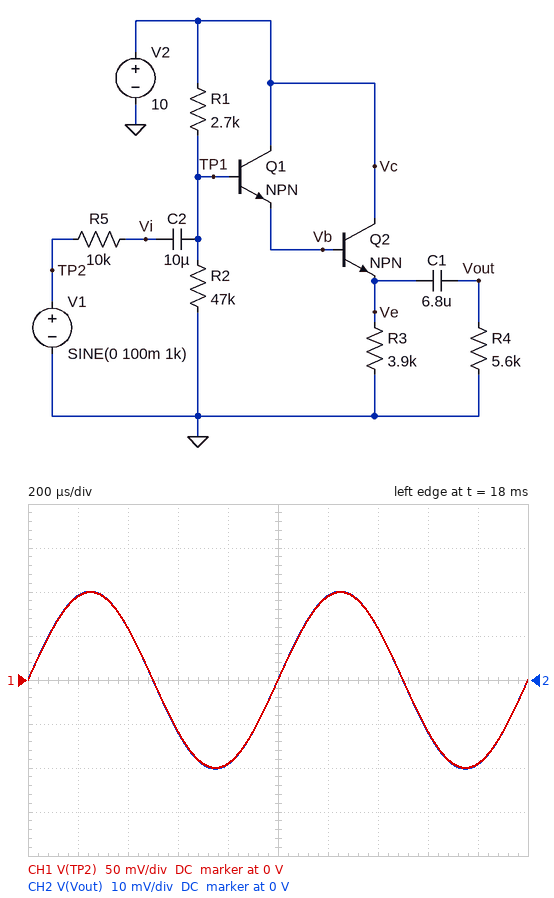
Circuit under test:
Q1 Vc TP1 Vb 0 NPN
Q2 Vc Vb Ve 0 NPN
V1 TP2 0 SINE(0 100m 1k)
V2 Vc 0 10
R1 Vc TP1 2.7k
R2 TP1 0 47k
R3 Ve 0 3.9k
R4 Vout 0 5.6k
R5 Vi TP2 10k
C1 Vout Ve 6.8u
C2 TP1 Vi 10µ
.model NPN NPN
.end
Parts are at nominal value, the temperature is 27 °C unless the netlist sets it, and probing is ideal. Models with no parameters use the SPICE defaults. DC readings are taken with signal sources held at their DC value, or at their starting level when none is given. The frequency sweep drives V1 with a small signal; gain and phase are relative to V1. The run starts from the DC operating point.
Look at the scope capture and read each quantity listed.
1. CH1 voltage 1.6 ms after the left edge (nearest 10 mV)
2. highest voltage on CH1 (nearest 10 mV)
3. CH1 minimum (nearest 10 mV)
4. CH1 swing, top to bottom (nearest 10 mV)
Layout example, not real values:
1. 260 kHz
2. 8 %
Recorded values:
1. -60 mV
2. 100 mV
3. -100 mV
4. 200 mV
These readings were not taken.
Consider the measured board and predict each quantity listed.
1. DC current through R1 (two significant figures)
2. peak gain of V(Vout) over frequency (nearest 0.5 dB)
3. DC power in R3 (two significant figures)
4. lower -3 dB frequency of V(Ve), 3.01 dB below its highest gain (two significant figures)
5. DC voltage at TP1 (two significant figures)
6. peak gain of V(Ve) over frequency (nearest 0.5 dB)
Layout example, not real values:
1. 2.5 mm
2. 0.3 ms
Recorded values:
1. 200 µA
2. -14.0 dB
3. 16 mW
4. 1.3 Hz
5. 9.5 V
6. -14.0 dB
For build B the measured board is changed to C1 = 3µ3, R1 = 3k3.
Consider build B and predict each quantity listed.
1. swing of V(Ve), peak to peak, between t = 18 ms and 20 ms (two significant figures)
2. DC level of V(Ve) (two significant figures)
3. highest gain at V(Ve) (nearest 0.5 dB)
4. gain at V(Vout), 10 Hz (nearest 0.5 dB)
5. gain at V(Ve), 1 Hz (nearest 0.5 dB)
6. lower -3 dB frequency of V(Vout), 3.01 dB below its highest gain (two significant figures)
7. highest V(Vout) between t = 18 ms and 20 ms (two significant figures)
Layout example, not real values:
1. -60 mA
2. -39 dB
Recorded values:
1. 47 mV
2. 7.9 V
3. -12.5 dB
4. -15.0 dB
5. -16.5 dB
6. 8.7 Hz
7. 23 mV
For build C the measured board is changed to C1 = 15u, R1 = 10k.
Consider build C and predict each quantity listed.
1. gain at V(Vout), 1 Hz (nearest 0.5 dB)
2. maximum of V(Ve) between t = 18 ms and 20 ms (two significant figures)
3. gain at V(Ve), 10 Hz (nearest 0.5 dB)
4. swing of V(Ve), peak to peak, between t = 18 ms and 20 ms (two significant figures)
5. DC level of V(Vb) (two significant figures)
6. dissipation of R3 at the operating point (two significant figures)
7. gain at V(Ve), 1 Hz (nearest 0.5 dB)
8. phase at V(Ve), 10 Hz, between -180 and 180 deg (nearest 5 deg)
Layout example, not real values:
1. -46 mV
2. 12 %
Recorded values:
1. -16.0 dB
2. 6.8 V
3. -7.0 dB
4. 89 mV
5. 7.6 V
6. 12 mW
7. -9.5 dB
8. 5 deg
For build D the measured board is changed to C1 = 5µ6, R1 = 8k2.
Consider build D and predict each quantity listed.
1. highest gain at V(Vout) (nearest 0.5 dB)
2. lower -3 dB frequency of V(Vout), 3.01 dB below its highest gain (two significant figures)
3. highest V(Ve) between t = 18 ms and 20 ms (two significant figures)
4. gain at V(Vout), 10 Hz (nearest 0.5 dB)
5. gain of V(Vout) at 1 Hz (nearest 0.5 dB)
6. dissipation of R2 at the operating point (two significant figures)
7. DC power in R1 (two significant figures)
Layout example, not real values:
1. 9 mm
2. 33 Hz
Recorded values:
1. -8.0 dB
2. 5.2 Hz
3. 7.1 V
4. -9.0 dB
5. -25.0 dB
6. 1.5 mW
7. 270 µW
